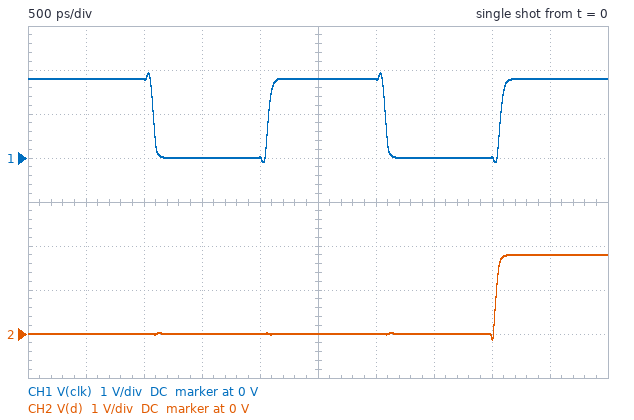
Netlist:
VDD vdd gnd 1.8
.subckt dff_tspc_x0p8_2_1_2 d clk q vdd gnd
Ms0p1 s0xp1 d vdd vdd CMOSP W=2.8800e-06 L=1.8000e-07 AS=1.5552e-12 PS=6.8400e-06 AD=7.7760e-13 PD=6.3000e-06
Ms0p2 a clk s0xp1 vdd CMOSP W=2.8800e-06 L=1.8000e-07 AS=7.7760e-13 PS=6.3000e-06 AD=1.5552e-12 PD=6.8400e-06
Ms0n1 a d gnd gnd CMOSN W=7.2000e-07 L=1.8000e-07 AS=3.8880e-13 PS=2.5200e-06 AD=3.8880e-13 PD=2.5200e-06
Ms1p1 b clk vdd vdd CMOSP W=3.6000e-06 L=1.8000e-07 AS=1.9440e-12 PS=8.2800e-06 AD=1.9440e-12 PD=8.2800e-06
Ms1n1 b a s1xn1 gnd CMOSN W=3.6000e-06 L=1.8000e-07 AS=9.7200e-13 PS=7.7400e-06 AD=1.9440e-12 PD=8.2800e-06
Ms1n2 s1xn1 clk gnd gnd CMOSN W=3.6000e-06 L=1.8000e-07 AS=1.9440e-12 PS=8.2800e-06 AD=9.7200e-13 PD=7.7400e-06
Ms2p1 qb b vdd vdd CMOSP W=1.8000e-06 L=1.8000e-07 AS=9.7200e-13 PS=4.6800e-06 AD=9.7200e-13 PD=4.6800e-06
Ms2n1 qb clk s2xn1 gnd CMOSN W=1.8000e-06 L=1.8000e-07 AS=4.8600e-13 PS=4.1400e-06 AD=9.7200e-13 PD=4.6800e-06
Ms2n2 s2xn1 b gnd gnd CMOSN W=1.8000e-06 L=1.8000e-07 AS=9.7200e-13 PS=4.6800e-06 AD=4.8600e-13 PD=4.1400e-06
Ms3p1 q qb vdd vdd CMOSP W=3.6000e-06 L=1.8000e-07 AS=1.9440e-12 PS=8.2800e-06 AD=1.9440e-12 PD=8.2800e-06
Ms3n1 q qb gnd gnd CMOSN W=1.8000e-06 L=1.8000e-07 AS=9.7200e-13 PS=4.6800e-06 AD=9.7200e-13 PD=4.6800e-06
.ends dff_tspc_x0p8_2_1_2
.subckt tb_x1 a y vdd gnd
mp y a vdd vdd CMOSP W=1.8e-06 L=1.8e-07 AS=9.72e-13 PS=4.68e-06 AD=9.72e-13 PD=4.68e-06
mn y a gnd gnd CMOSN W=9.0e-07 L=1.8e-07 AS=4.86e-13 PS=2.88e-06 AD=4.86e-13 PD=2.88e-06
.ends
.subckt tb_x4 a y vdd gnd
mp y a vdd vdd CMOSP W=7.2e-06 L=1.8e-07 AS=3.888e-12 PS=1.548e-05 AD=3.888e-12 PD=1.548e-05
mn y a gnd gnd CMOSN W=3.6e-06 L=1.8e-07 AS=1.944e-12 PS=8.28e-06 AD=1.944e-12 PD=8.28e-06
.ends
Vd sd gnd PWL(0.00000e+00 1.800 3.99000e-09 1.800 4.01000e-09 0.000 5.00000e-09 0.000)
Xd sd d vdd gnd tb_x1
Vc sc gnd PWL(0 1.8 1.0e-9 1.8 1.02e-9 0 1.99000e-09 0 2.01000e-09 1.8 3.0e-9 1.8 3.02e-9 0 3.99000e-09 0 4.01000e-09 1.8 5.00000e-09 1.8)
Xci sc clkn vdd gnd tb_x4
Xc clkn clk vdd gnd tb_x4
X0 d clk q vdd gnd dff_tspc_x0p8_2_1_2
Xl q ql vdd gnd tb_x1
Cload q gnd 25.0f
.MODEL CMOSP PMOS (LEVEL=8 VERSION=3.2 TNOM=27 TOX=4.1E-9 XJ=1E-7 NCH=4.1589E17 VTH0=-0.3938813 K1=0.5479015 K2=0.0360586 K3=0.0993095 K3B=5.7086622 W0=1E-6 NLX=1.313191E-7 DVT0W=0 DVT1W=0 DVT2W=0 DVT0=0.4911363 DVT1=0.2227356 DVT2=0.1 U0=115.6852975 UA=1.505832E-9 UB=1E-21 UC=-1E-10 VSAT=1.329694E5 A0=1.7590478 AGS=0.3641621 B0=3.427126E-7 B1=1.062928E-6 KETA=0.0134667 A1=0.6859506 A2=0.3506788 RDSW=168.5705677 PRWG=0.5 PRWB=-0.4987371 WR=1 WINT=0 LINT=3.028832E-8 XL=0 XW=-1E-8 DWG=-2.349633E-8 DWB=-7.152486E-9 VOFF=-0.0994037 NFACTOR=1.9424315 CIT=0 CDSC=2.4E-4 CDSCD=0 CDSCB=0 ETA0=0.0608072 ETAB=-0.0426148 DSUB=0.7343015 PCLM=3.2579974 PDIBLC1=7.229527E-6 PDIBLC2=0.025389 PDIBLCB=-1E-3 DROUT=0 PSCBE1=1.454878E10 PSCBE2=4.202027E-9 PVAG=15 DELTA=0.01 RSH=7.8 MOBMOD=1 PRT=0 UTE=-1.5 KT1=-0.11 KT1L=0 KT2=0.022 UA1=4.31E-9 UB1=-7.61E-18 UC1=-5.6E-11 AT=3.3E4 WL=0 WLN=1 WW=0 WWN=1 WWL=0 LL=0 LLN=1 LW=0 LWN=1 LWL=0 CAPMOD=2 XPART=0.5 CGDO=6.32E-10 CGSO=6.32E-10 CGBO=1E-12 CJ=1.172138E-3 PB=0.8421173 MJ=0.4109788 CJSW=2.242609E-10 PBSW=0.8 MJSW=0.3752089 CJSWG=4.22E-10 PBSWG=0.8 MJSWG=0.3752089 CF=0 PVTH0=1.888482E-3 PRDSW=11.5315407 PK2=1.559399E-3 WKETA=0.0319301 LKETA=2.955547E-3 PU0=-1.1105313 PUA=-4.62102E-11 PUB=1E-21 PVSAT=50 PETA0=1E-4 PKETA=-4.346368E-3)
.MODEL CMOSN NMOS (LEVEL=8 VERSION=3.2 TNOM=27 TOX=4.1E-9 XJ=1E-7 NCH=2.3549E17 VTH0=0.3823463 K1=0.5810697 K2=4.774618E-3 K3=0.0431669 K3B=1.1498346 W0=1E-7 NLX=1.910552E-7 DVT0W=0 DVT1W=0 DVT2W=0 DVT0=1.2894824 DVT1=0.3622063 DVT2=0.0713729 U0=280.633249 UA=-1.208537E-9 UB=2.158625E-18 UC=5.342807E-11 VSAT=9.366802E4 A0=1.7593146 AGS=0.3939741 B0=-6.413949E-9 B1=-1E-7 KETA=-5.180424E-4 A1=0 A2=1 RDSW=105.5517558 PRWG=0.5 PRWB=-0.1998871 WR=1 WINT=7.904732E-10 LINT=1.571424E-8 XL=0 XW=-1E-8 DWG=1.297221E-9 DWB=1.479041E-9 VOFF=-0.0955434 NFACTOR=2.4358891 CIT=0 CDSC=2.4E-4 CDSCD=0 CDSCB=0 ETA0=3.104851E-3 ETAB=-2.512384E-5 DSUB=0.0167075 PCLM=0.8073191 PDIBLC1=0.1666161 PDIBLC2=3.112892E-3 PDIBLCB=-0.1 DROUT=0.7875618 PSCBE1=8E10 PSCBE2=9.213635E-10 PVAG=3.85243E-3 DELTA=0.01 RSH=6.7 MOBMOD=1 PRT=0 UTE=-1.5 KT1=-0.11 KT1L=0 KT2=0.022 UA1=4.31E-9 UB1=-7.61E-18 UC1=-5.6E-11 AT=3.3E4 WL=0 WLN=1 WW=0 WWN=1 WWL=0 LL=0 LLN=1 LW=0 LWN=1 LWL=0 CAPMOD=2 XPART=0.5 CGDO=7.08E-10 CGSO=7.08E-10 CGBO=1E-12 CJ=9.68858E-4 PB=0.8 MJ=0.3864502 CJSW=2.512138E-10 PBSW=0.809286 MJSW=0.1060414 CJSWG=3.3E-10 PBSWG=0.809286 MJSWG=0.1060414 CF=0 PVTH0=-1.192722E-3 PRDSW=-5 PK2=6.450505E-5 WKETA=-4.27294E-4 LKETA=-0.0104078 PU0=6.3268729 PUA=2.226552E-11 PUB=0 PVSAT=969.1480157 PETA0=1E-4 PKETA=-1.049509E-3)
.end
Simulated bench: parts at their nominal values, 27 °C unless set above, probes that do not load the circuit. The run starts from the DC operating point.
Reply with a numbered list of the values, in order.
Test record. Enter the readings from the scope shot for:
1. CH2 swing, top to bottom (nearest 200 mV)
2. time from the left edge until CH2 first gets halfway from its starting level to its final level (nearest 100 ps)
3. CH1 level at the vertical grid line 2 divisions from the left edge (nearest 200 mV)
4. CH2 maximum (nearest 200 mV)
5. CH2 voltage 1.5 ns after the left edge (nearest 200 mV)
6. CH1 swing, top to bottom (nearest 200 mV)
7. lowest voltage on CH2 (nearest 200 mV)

1. 2.0 V
2. 4.0 ns
3. 1.8 V
4. 1.8 V
5. 0 V
6. 2.0 V
7. -200 mV
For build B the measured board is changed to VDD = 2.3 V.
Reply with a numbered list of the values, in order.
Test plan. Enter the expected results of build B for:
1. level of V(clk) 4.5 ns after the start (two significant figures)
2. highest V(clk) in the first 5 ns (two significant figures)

1. 2.3 V
2. 2.4 V
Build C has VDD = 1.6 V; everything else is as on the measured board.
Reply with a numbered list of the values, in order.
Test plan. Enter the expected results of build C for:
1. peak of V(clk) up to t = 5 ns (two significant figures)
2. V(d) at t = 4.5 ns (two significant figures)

1. 1.7 V
2. 1.6 V
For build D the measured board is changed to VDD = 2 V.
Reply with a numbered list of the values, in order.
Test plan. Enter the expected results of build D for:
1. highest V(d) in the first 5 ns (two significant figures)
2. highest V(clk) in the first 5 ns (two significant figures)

1. 2.0 V
2. 2.1 V
